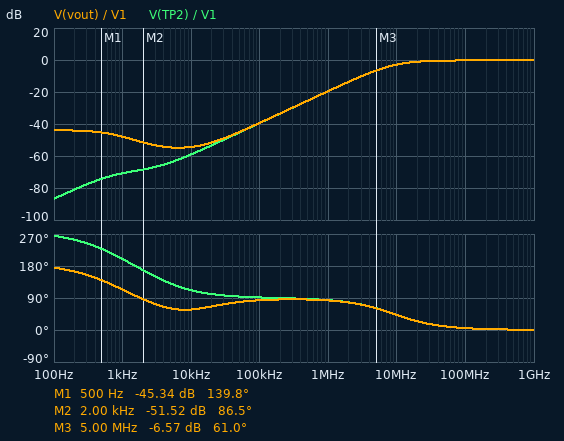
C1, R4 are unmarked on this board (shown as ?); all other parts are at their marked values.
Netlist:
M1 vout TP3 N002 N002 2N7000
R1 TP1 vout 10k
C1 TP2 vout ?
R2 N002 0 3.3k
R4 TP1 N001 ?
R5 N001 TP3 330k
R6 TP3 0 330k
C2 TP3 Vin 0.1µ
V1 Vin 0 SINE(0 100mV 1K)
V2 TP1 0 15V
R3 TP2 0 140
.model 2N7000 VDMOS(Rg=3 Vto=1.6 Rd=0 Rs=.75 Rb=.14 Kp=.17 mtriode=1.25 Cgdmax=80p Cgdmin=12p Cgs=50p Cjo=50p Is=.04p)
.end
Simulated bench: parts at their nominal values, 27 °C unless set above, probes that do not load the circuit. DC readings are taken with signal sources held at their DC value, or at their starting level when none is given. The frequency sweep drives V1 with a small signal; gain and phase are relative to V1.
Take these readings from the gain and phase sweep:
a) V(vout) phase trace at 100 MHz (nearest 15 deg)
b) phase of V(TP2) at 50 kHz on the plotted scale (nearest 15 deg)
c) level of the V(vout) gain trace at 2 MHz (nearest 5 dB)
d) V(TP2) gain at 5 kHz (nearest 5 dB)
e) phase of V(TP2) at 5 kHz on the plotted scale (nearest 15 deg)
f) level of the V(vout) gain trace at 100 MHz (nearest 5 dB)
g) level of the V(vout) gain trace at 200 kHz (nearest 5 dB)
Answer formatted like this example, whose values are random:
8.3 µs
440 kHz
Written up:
0 deg
90 deg
-15 dB
-65 dB
135 deg
0 dB
-35 dB
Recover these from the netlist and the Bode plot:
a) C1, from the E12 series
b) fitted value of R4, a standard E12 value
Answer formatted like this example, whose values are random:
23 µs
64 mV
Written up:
82 nF
150 kΩ
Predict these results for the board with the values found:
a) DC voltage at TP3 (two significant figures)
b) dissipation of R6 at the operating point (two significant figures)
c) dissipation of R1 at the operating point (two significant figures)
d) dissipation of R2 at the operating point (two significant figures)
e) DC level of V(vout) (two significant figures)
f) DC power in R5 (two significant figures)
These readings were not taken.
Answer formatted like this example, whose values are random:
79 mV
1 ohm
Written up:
6.1 V
110 µW
13 mW
4.2 mW
3.7 V
110 µW
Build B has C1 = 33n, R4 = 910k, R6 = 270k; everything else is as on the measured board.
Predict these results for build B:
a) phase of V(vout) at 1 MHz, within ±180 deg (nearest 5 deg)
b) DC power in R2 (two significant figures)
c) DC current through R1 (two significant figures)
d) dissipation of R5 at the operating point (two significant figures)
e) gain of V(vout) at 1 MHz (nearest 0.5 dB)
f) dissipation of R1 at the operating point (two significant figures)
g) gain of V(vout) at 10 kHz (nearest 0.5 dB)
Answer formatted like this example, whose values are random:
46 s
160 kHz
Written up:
155 deg
360 µW
330 µA
33 µW
-27.5 dB
1.1 mW
-17.0 dB
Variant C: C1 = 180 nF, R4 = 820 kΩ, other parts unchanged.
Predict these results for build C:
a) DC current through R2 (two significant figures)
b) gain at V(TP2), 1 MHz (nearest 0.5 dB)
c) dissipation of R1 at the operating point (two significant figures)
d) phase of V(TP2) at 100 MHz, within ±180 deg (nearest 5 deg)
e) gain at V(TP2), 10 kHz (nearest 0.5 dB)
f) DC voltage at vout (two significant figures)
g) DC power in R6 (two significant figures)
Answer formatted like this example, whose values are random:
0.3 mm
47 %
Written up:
520 µA
-27.0 dB
2.7 mW
25 deg
-28.0 dB
9.8 V
34 µW
